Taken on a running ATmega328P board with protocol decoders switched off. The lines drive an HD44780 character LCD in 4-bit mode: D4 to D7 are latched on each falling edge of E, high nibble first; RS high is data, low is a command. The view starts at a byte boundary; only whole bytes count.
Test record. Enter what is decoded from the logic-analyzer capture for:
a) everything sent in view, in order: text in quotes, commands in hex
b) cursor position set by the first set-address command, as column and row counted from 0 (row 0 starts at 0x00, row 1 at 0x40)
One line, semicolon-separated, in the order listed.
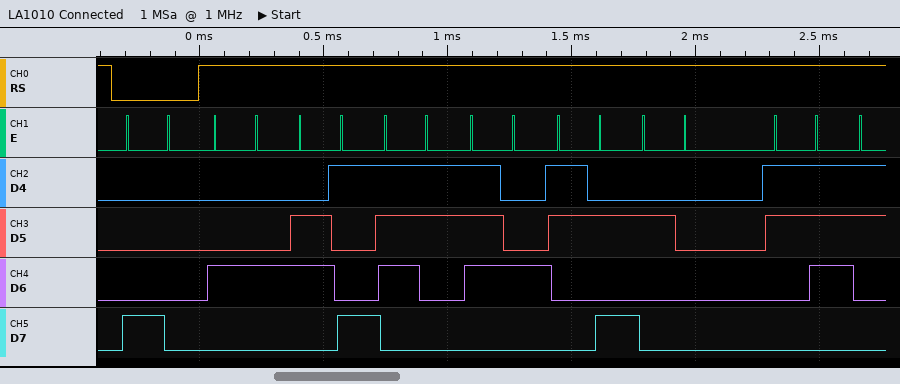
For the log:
0x80 "Dist: 7"; column 0, row 0
